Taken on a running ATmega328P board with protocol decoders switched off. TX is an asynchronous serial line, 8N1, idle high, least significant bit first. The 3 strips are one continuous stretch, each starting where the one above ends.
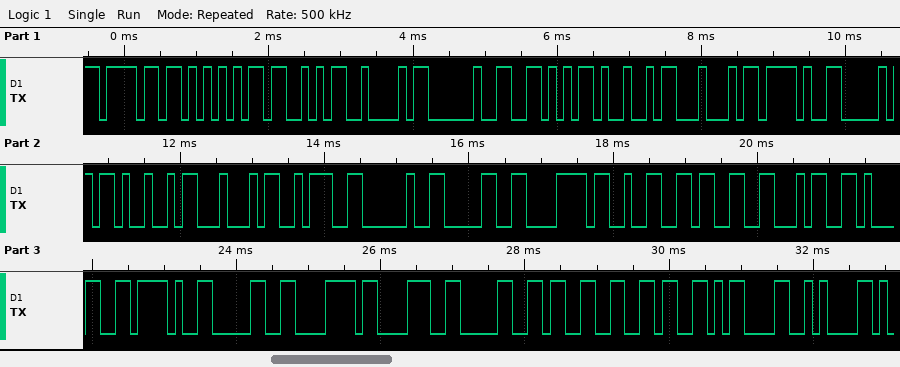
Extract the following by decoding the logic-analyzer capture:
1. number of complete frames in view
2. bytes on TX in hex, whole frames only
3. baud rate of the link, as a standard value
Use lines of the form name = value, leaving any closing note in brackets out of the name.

number of complete frames in view = 29
bytes on TX in hex, whole frames only = 6F 55 53 42 20 56 49 44 2F 50 49 44 3A 20 30 78 32 33 34 31 2F 30 78 38 30 33 36 0D 0A
baud rate of the link, as a standard value = 9600 baud
